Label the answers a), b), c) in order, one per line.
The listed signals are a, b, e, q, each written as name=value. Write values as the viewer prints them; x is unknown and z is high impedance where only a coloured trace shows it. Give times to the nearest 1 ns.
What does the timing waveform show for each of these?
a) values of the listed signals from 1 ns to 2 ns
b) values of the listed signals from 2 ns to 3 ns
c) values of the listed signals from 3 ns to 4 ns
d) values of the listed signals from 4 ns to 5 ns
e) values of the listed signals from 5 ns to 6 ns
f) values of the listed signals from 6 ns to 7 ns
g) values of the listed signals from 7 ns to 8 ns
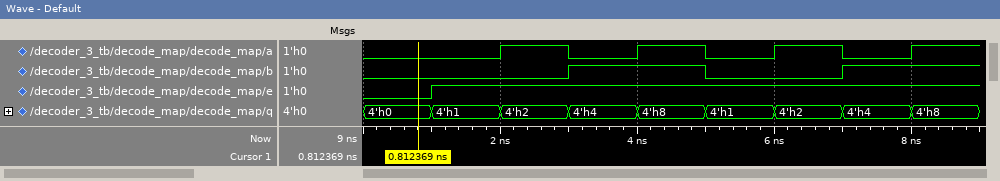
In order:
a) a=0, b=0, e=1, q=4'h1
b) a=1, b=0, e=1, q=4'h2
c) a=0, b=1, e=1, q=4'h4
d) a=1, b=1, e=1, q=4'h8
e) a=0, b=0, e=1, q=4'h1
f) a=1, b=0, e=1, q=4'h2
g) a=0, b=1, e=1, q=4'h4
